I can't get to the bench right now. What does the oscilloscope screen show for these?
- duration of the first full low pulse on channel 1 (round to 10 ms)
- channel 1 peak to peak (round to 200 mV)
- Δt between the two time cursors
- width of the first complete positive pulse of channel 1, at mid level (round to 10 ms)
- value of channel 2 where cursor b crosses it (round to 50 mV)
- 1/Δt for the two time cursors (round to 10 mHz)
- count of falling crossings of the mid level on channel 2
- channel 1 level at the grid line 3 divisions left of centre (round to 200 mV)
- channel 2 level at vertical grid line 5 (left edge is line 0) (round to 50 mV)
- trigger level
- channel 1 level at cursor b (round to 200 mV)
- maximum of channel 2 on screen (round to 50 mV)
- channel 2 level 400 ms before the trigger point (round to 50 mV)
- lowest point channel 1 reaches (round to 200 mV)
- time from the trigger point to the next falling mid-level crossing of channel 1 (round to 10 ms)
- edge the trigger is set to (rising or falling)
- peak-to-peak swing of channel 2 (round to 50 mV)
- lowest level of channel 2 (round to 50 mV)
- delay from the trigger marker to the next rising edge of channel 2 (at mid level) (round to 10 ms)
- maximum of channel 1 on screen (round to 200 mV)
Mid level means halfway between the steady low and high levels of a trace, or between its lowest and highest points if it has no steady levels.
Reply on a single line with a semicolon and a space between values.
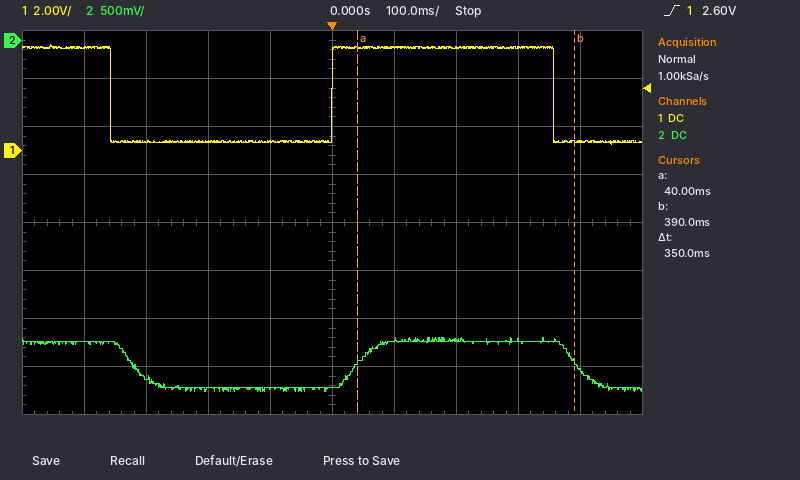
360 ms; 4.2 V; 350 ms; 360 ms; -3.35 V; 2.86 Hz; 2; 400 mV; -3.60 V; 2.60 V; 400 mV; -3.10 V; -3.15 V; 200 mV; 360 ms; rising; 550 mV; -3.65 V; 40 ms; 4.4 V
